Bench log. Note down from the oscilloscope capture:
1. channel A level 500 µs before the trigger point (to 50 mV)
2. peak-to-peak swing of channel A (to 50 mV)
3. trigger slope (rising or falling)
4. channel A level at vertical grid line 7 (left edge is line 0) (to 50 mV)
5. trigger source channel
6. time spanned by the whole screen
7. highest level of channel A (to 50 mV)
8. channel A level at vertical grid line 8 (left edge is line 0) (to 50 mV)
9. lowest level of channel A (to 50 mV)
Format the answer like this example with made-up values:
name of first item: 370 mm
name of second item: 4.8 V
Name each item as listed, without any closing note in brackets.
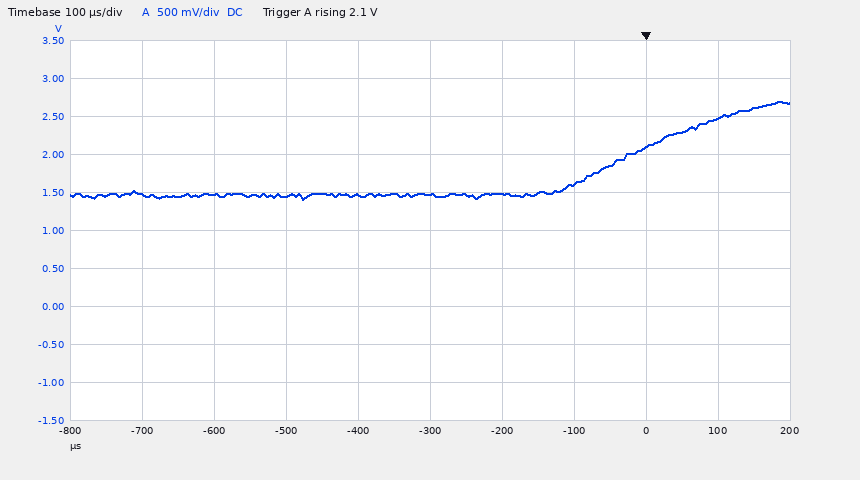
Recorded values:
channel A level 500 µs before the trigger point: 1.45 V
peak-to-peak swing of channel A: 1.30 V
trigger slope: rising
channel A level at vertical grid line 7 (left edge is line 0): 1.60 V
trigger source channel: channel A
time spanned by the whole screen: 1 ms
highest level of channel A: 2.70 V
channel A level at vertical grid line 8 (left edge is line 0): 2.10 V
lowest level of channel A: 1.40 V
